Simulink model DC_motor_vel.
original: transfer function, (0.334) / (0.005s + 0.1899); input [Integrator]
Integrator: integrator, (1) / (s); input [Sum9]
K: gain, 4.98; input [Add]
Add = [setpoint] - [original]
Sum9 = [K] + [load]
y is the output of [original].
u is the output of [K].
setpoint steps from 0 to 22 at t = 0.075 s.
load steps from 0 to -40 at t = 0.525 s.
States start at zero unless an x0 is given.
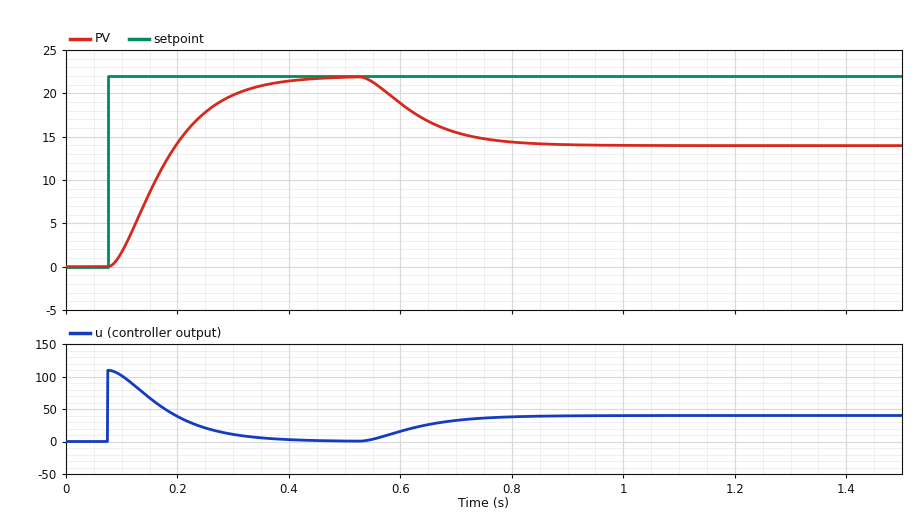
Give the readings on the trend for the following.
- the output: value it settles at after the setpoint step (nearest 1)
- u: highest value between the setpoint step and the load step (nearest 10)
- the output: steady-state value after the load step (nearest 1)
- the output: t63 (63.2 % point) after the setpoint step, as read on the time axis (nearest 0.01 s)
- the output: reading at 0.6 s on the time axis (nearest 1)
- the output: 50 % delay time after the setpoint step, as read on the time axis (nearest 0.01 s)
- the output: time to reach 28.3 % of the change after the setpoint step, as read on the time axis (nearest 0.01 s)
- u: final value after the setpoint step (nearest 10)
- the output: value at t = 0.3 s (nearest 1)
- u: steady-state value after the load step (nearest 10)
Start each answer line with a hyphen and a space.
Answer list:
- 22
- 110
- 14
- 0.20 s
- 19
- 0.17 s
- 0.13 s
- 0
- 20
- 40
